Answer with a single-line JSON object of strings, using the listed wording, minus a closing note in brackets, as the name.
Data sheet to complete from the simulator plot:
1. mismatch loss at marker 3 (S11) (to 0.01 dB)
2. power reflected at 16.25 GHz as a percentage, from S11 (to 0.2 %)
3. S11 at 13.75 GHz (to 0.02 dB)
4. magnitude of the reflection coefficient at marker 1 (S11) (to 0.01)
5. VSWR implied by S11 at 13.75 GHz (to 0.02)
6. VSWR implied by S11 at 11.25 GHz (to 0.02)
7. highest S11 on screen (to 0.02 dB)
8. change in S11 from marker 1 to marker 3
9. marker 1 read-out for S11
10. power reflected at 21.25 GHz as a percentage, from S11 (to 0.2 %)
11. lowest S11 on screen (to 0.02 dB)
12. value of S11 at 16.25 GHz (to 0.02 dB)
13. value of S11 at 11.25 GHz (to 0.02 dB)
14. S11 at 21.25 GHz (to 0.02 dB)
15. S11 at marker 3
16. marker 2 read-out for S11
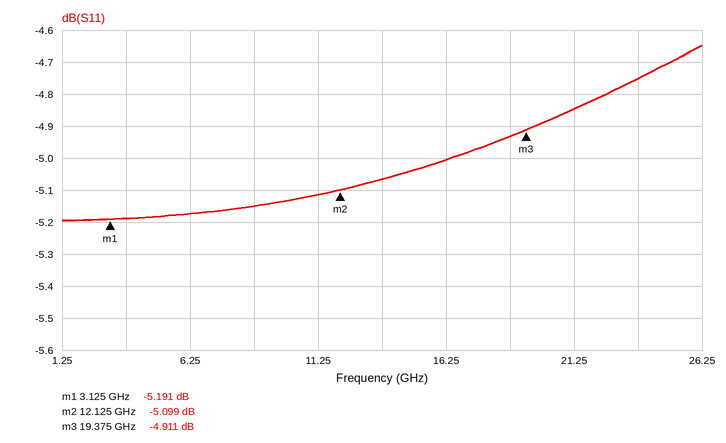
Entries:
{"mismatch loss at marker 3 (S11)": "1.69 dB", "power reflected at 16.25 GHz as a percentage, from S11": "31.6 %", "S11 at 13.75 GHz": "-5.06 dB", "magnitude of the reflection coefficient at marker 1 (S11)": "0.55", "VSWR implied by S11 at 13.75 GHz": "3.52", "VSWR implied by S11 at 11.25 GHz": "3.50", "highest S11 on screen": "-4.64 dB", "change in S11 from marker 1 to marker 3": "0.280 dB", "marker 1 read-out for S11": "-5.191 dB", "power reflected at 21.25 GHz as a percentage, from S11": "32.8 %", "lowest S11 on screen": "-5.20 dB", "value of S11 at 16.25 GHz": "-5.00 dB", "value of S11 at 11.25 GHz": "-5.12 dB", "S11 at 21.25 GHz": "-4.84 dB", "S11 at marker 3": "-4.911 dB", "marker 2 read-out for S11": "-5.099 dB"}
